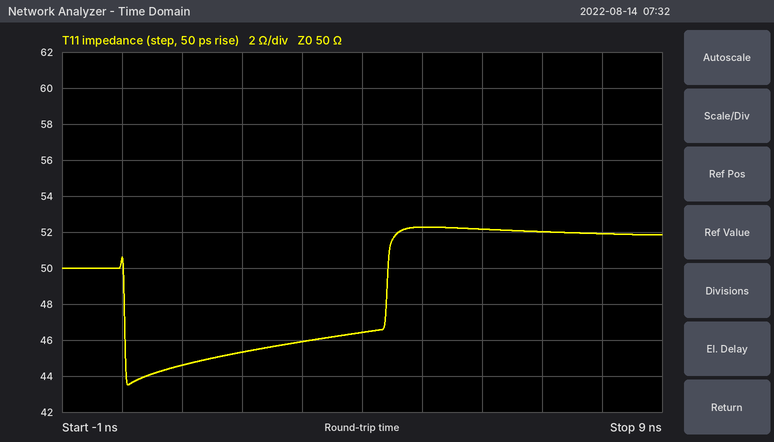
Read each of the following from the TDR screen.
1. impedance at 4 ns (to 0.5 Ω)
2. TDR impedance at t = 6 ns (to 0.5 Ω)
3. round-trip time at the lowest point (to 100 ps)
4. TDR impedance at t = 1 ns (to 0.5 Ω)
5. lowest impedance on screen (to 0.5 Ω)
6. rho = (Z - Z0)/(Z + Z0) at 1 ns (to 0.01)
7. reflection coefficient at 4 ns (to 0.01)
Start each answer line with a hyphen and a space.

- 46.5 Ω
- 52.0 Ω
- 100 ps
- 44.5 Ω
- 43.5 Ω
- -0.06
- -0.04
